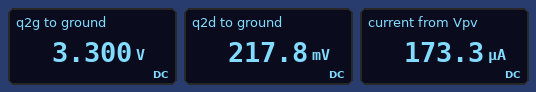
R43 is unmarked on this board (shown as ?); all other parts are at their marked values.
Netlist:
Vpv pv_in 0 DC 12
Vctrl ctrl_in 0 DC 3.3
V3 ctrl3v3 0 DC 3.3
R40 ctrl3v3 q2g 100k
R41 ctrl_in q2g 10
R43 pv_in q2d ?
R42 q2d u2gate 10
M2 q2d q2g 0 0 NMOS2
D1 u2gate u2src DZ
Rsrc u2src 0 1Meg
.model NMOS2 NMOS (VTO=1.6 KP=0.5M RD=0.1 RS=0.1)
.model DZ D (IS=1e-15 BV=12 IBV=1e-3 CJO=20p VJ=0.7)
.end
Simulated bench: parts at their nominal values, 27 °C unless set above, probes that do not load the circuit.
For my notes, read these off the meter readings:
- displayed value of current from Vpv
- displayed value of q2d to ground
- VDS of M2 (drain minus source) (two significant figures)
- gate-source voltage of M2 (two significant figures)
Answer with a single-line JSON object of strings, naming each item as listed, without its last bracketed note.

{"displayed value of current from Vpv": "173.3 µA", "displayed value of q2d to ground": "217.8 mV", "VDS of M2 (drain minus source)": "220 mV", "gate-source voltage of M2": "3.3 V"}
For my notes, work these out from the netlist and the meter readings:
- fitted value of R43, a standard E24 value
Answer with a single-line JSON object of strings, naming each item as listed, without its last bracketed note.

{"fitted value of R43, a standard E24 value": "68 kΩ"}
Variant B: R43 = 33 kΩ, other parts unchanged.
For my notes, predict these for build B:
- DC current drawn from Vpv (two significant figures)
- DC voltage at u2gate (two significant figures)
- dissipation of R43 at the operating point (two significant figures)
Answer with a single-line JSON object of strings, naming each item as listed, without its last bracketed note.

{"DC current drawn from Vpv": "350 µA", "DC voltage at u2gate": "480 mV", "dissipation of R43 at the operating point": "4.0 mW"}
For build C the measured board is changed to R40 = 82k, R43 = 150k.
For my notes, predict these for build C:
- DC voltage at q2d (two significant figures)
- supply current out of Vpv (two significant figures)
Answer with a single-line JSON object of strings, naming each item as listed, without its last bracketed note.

{"DC voltage at q2d": "96 mV", "supply current out of Vpv": "79 µA"}
